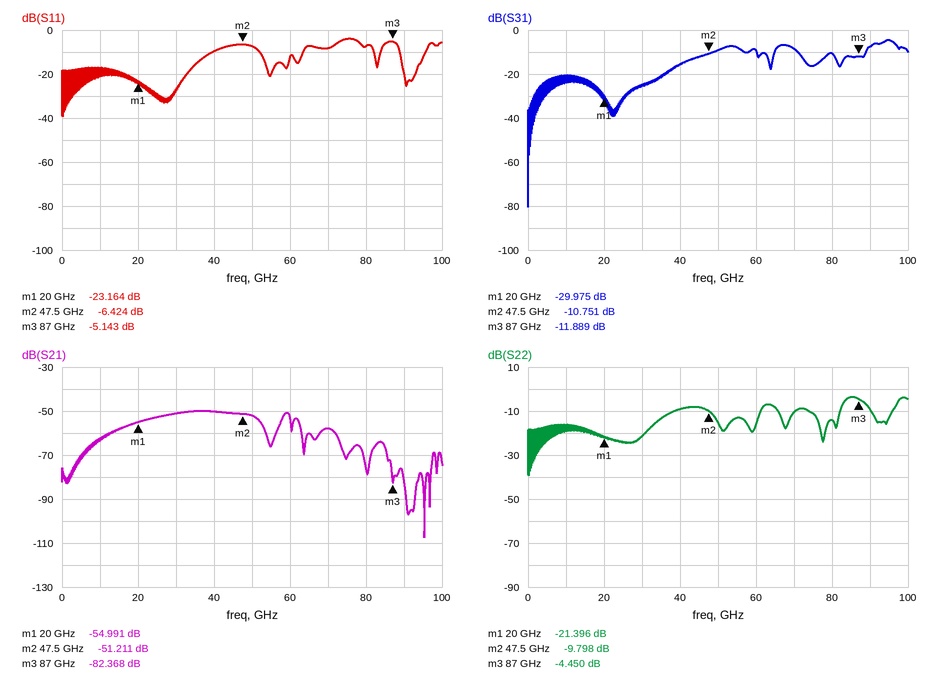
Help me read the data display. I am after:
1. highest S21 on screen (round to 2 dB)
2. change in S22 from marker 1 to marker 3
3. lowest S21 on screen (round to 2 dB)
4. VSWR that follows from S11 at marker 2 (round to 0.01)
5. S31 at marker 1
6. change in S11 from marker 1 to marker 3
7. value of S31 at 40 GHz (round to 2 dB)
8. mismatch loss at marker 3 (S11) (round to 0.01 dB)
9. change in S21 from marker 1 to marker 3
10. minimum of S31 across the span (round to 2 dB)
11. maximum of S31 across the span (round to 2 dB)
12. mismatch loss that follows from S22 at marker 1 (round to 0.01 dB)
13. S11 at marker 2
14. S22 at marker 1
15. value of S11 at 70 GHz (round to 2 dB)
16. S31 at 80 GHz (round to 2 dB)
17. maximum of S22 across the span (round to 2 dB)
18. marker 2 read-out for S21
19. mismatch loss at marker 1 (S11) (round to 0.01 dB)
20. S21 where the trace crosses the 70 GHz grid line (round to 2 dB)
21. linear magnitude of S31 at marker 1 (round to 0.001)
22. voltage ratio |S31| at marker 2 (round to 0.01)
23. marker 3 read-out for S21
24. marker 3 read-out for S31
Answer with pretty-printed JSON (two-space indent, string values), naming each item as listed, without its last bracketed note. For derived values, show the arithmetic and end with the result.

{
  "highest S21 on screen": "-50 dB",
  "change in S22 from marker 1 to marker 3": "-4.45 − (-21.396) = 16.946 dB",
  "lowest S21 on screen": "-108 dB",
  "VSWR that follows from S11 at marker 2": "(1 + 0.4773)/(1 − 0.4773) ≈ 2.83",
  "S31 at marker 1": "-29.975 dB",
  "change in S11 from marker 1 to marker 3": "-5.143 − (-23.164) = 18.021 dB",
  "value of S31 at 40 GHz": "-16 dB",
  "mismatch loss at marker 3 (S11)": "−10 log10(1 − 10^(-5.143/10)) ≈ 1.59 dB",
  "change in S21 from marker 1 to marker 3": "-82.368 − (-54.991) = -27.377 dB",
  "minimum of S31 across the span": "-80 dB",
  "maximum of S31 across the span": "-4 dB",
  "mismatch loss that follows from S22 at marker 1": "−10 log10(1 − 10^(-21.396/10)) ≈ 0.03 dB",
  "S11 at marker 2": "-6.424 dB",
  "S22 at marker 1": "-21.396 dB",
  "value of S11 at 70 GHz": "-8 dB",
  "S31 at 80 GHz": "-10 dB",
  "maximum of S22 across the span": "-4 dB",
  "marker 2 read-out for S21": "-51.211 dB",
  "mismatch loss at marker 1 (S11)": "−10 log10(1 − 10^(-23.164/10)) ≈ 0.02 dB",
  "S21 where the trace crosses the 70 GHz grid line": "-58 dB",
  "linear magnitude of S31 at marker 1": "10^(-29.975/20) ≈ 0.032",
  "voltage ratio |S31| at marker 2": "10^(-10.751/20) ≈ 0.29",
  "marker 3 read-out for S21": "-82.368 dB",
  "marker 3 read-out for S31": "-11.889 dB"
}
